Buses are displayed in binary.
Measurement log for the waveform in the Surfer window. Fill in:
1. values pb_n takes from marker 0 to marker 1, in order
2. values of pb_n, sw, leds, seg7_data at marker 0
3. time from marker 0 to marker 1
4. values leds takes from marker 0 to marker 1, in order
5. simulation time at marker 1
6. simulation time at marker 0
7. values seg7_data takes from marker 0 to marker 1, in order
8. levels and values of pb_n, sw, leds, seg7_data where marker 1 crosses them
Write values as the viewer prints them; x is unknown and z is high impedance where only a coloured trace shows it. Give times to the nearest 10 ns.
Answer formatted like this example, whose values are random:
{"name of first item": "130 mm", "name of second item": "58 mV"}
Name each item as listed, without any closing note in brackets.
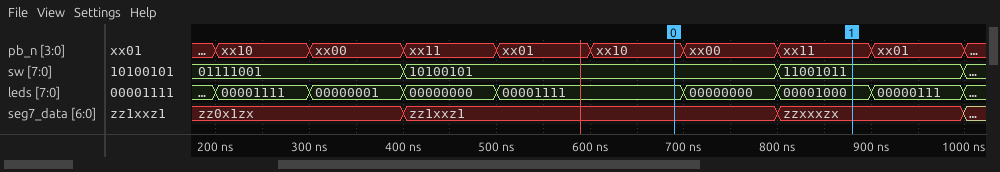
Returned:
{"values pb_n takes from marker 0 to marker 1, in order": "xx10, xx00, xx11", "values of pb_n, sw, leds, seg7_data at marker 0": "pb_n=xx10, sw=10100101, leds=00001111, seg7_data=zz1xxz1", "time from marker 0 to marker 1": "190 ns", "values leds takes from marker 0 to marker 1, in order": "00001111, 00000000, 00001000", "simulation time at marker 1": "880 ns", "simulation time at marker 0": "690 ns", "values seg7_data takes from marker 0 to marker 1, in order": "zz1xxz1, zzxxxzx", "levels and values of pb_n, sw, leds, seg7_data where marker 1 crosses them": "pb_n=xx11, sw=11001011, leds=00001000, seg7_data=zzxxxzx"}
